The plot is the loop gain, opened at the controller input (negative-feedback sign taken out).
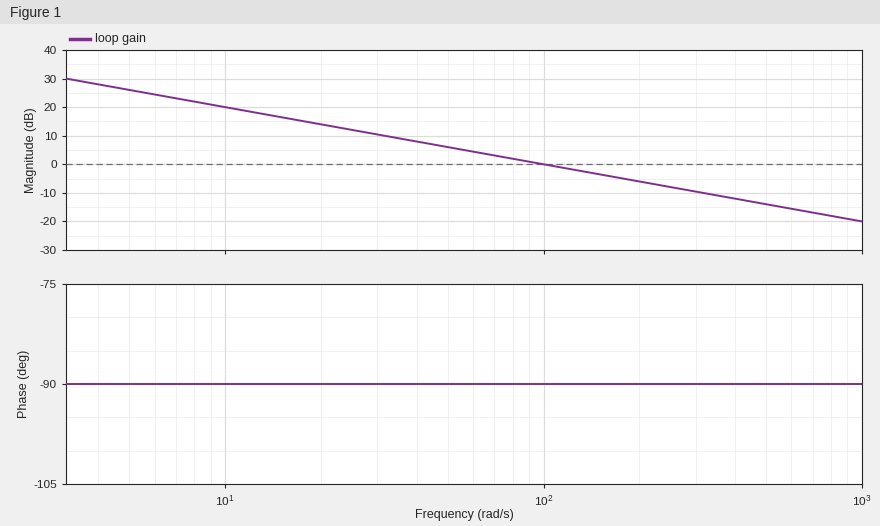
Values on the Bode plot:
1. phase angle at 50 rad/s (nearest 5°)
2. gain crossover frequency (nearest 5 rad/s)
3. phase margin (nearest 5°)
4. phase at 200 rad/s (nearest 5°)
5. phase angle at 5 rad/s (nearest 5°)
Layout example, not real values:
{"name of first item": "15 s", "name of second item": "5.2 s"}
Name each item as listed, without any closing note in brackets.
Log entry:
{"phase angle at 50 rad/s": "-90°", "gain crossover frequency": "100 rad/s", "phase margin": "90°", "phase at 200 rad/s": "-90°", "phase angle at 5 rad/s": "-90°"}
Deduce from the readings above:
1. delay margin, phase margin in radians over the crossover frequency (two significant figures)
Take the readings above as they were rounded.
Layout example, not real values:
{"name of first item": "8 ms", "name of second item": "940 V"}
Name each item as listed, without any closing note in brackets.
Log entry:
{"delay margin, phase margin in radians over the crossover frequency": "0.016 s"}
